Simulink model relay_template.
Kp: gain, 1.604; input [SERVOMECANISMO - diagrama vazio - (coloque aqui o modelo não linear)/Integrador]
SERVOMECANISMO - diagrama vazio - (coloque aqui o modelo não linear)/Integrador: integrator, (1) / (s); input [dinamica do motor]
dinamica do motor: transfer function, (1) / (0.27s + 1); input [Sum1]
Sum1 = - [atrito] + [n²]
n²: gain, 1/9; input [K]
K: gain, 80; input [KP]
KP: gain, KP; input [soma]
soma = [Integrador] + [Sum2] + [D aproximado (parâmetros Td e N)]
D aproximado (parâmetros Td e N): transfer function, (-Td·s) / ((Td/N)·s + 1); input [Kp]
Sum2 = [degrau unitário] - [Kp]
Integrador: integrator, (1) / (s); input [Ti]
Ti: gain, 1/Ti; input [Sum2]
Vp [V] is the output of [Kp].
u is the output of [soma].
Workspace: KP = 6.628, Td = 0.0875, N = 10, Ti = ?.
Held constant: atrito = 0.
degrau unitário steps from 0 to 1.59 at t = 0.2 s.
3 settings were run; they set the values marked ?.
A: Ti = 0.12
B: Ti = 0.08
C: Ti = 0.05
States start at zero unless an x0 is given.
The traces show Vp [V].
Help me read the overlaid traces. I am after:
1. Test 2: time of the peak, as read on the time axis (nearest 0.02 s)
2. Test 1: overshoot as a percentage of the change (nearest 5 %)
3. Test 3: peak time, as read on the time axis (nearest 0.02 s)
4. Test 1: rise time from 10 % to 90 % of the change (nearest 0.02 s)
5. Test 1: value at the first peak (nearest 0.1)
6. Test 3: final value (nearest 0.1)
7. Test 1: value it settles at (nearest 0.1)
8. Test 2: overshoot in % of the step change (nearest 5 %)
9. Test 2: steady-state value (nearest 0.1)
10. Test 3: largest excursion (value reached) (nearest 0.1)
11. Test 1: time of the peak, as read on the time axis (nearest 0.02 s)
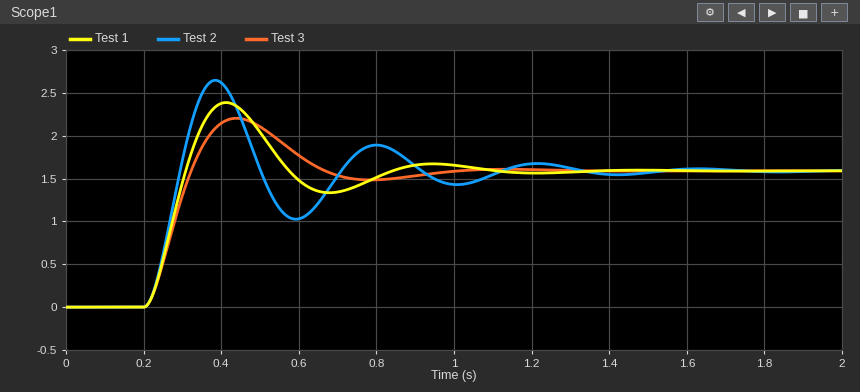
0.38 s
50 %
0.44 s
0.08 s
2.4
1.6
1.6
65 %
1.6
2.2
0.42 s
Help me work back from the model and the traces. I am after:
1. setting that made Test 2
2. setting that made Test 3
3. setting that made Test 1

C
A
B
